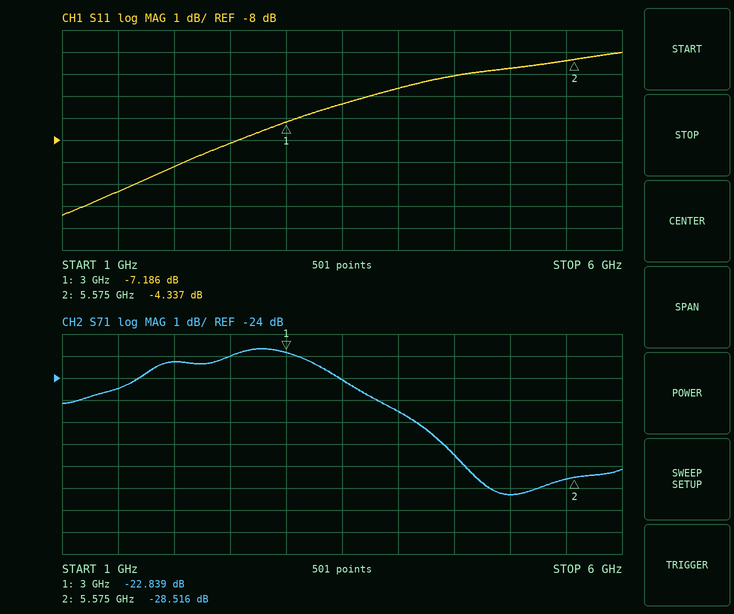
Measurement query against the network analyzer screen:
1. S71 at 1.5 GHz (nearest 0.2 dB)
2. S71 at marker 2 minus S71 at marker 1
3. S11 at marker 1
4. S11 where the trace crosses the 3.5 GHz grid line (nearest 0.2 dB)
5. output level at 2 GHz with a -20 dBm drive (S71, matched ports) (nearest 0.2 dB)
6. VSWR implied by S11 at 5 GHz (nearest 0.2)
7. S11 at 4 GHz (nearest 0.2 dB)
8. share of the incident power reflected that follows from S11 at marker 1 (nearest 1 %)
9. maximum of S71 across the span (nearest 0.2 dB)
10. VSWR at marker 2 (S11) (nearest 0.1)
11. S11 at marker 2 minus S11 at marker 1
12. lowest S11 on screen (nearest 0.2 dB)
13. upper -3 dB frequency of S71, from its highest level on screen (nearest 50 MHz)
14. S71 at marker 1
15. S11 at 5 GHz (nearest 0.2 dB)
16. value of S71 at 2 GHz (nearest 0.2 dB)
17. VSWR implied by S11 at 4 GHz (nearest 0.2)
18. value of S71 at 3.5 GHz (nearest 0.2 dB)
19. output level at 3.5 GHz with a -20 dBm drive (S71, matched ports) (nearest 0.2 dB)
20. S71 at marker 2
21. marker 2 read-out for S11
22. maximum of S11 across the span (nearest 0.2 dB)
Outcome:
-24.4 dB
-5.677 dB
-7.186 dB
-6.4 dB
-43.2 dBm
3.8
-5.6 dB
19 %
-22.6 dB
4.1
2.849 dB
-11.4 dB
4.05 GHz
-22.839 dB
-4.8 dB
-23.2 dB
3.2
-24.0 dB
-44.0 dBm
-28.516 dB
-4.337 dB
-4.0 dB
